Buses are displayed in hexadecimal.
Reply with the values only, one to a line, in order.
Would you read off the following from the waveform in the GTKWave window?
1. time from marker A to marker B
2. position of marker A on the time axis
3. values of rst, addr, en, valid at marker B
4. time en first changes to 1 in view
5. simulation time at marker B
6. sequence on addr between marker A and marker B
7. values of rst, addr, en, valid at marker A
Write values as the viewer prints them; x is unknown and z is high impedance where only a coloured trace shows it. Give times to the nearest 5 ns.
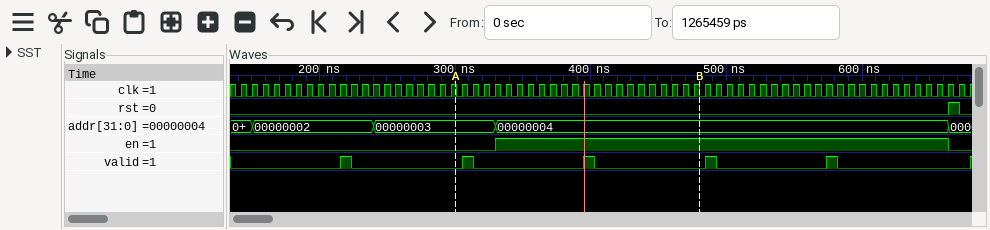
180 ns
300 ns
rst=0, addr=00000004, en=1, valid=0
330 ns
480 ns
00000003, 00000004
rst=0, addr=00000003, en=0, valid=0
